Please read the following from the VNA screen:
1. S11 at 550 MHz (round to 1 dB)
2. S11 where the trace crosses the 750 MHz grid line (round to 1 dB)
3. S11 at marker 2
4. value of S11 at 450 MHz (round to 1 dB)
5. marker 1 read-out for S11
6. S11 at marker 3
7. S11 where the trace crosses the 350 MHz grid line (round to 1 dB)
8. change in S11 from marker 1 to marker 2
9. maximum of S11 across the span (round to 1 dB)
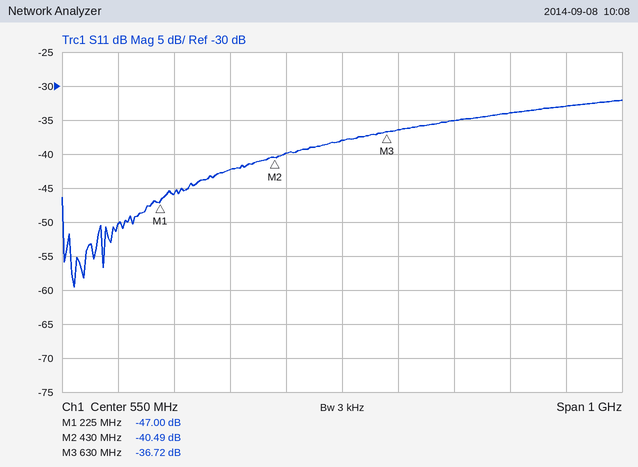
-38 dB
-35 dB
-40.49 dB
-40 dB
-47.00 dB
-36.72 dB
-42 dB
6.51 dB
-32 dB
